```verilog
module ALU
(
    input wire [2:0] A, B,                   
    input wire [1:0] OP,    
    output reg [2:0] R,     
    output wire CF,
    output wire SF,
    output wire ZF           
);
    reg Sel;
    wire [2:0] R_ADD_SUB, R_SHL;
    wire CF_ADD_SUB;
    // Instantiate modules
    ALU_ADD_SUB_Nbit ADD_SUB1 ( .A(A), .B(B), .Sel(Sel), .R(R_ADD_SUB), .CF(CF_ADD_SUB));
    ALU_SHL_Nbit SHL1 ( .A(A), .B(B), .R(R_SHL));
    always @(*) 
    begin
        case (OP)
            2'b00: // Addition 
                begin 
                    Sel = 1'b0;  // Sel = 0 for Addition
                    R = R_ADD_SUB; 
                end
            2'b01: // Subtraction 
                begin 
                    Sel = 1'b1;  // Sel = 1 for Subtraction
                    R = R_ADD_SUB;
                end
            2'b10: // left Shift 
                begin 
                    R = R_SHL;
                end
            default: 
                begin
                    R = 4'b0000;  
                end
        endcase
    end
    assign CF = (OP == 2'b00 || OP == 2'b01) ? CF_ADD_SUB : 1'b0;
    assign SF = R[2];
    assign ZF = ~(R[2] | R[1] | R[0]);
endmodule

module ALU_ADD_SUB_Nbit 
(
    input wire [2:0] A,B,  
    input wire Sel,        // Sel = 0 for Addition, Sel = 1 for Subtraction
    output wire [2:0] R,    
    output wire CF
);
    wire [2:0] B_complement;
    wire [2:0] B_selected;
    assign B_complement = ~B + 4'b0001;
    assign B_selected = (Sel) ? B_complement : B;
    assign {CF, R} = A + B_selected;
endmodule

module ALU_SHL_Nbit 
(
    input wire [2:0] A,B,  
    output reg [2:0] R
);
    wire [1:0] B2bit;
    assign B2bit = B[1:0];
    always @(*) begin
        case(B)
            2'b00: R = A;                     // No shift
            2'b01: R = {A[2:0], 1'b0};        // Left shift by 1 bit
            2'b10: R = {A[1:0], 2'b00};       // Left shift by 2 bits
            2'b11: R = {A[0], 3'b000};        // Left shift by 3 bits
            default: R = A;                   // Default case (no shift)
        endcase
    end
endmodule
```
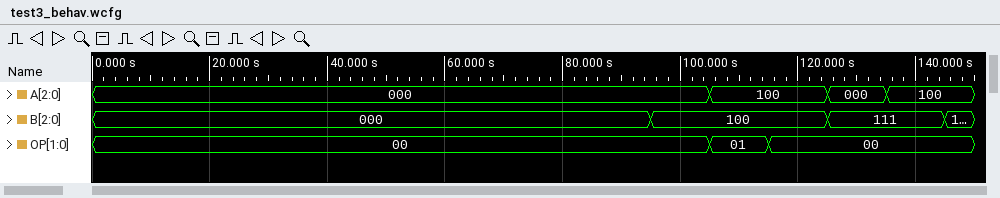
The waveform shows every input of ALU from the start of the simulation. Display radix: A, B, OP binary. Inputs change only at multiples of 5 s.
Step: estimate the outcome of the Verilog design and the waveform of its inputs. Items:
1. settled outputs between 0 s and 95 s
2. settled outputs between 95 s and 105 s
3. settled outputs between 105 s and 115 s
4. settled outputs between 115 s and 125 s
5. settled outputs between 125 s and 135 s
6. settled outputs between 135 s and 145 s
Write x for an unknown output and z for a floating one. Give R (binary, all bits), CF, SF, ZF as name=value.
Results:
R=000, CF=0, SF=0, ZF=1
R=100, CF=0, SF=1, ZF=0
R=000, CF=1, SF=0, ZF=1
R=000, CF=1, SF=0, ZF=1
R=111, CF=0, SF=1, ZF=0
R=011, CF=1, SF=0, ZF=0
